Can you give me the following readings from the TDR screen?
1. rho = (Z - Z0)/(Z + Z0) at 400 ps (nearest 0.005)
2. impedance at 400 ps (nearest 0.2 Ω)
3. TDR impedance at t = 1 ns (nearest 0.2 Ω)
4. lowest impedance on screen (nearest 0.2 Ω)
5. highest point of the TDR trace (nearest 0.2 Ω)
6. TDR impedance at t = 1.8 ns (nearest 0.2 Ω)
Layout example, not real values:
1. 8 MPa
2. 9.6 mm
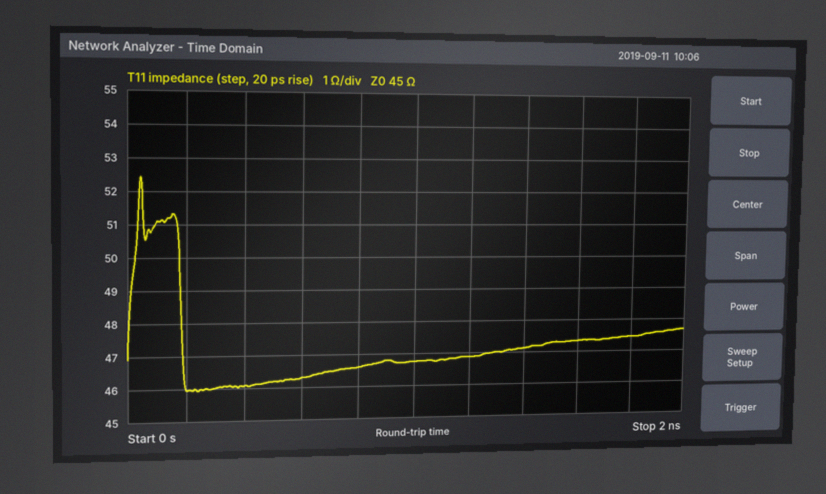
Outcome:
1. +0.010
2. 46.0 Ω
3. 46.8 Ω
4. 46.0 Ω
5. 52.4 Ω
6. 47.4 Ω
